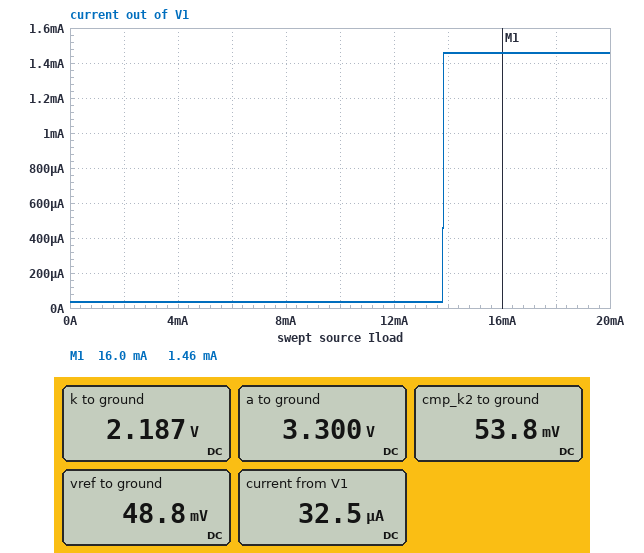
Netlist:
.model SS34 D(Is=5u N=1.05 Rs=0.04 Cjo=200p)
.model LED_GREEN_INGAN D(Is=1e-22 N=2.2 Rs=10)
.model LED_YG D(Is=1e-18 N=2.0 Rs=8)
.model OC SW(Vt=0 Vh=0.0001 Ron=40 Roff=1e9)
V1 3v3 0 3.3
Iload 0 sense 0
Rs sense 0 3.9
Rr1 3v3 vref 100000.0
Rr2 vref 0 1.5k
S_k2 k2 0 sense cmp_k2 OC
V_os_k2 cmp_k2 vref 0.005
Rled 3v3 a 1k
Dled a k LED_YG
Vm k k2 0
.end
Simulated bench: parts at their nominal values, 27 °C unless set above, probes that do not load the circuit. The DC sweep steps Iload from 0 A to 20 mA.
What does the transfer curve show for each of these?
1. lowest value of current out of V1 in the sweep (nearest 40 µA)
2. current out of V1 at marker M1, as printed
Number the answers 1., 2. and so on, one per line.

1. 40 µA
2. 1.46 mA
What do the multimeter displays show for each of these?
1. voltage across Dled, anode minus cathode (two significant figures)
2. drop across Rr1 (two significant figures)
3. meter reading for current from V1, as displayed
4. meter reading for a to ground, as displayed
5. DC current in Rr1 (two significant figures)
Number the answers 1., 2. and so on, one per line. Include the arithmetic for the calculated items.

1. 3.3 V - 2.187 V = 1.1 V
2. 3.3 V - 48.8 mV = 3.3 V
3. 32.5 µA
4. 3.300 V
5. (3.3 V - 48.8 mV) / 100 kΩ = 33 µA
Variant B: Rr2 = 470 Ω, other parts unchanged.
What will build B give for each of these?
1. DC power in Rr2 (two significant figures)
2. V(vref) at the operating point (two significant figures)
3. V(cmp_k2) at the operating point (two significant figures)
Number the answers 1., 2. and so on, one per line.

1. 510 nW
2. 15 mV
3. 20 mV
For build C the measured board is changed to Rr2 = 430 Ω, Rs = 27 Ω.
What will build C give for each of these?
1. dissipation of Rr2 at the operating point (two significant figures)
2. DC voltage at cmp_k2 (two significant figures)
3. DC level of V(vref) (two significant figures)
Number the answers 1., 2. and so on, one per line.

1. 460 nW
2. 19 mV
3. 14 mV
